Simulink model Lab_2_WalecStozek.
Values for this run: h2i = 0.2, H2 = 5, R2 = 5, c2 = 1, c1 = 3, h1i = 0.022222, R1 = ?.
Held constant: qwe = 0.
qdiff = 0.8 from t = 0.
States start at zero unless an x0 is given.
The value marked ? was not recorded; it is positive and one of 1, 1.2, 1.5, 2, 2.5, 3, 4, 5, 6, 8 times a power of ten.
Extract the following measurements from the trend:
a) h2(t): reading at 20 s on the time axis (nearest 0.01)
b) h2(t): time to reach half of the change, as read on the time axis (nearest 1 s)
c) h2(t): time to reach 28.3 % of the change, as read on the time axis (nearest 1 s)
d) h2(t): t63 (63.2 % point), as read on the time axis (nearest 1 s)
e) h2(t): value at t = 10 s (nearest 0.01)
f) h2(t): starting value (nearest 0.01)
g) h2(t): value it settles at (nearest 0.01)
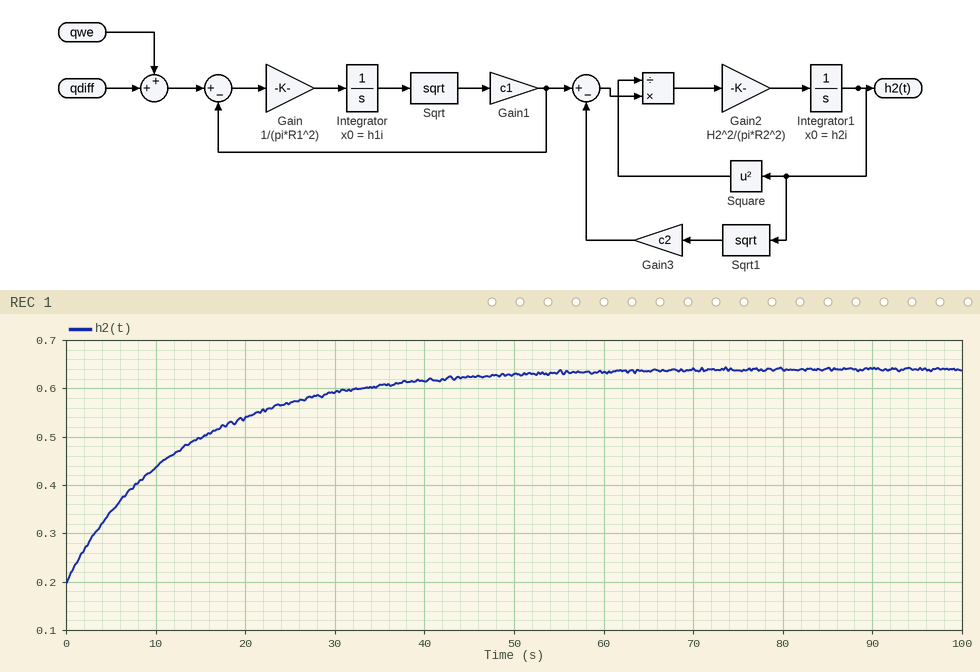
0.54
9 s
4 s
13 s
0.44
0.20
0.64
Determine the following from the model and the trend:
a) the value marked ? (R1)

5
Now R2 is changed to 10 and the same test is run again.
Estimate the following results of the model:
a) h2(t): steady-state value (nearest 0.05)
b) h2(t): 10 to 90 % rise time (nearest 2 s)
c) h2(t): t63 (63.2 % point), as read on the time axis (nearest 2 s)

0.65
36 s
16 s
